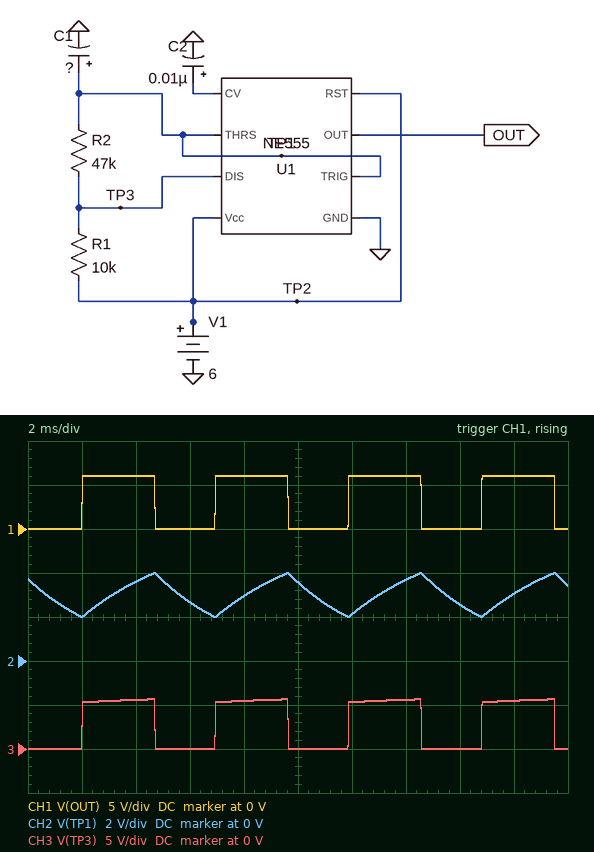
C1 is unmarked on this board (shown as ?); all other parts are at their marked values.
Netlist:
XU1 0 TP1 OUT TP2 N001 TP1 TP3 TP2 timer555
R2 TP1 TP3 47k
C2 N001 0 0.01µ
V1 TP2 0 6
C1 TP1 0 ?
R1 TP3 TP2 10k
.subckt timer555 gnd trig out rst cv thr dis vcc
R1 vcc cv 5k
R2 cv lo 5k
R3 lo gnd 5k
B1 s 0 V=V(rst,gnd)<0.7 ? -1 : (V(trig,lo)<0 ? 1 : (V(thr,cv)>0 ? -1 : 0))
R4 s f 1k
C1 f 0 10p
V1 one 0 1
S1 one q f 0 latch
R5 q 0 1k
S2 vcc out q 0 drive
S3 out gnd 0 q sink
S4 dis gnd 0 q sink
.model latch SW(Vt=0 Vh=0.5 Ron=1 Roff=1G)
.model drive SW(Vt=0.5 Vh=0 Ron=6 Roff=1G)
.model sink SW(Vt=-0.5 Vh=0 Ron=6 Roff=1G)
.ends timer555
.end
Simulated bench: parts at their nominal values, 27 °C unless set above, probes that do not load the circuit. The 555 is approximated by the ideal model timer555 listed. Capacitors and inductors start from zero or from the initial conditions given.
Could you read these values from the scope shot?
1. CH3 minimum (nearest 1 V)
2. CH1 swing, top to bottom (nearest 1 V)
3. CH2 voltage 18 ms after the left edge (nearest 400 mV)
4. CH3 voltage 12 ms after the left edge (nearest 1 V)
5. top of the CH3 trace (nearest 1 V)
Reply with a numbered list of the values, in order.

1. 0 V
2. 6 V
3. 3.2 V
4. 5 V
5. 6 V
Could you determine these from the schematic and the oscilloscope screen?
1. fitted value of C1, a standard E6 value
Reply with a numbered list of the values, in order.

1. 68 nF
